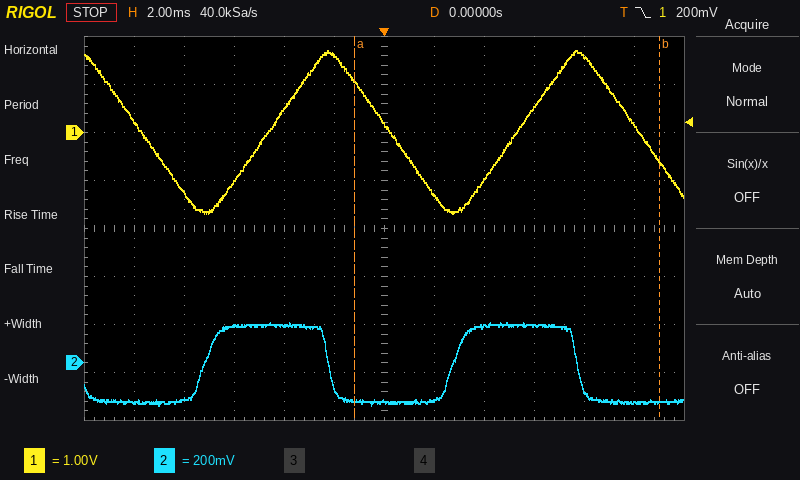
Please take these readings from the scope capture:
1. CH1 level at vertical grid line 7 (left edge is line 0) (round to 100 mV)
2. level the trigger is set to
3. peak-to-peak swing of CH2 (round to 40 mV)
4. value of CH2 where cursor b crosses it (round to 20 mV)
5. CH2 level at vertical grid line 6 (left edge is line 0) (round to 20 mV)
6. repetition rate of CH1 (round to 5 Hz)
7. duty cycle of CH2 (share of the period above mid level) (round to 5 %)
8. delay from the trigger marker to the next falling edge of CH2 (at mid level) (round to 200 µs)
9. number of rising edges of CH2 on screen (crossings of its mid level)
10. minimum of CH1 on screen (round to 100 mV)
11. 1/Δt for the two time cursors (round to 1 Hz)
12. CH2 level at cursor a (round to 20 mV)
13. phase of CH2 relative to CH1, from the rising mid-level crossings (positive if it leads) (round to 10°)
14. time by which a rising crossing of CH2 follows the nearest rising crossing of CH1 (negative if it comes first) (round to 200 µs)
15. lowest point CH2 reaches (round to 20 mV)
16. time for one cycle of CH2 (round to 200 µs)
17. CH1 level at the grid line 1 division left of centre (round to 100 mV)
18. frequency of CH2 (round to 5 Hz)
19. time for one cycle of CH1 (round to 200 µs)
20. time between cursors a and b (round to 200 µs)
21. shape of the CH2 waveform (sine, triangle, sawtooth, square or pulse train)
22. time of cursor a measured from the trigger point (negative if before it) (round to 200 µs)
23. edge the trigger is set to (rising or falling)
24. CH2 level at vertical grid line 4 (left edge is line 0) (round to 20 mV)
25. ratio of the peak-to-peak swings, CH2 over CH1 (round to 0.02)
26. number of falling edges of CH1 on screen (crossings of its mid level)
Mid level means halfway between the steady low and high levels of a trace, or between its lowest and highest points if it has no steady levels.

-1.3 V
200 mV
360 mV
-160 mV
-160 mV
100 Hz
50 %
7.8 ms
2
-1.7 V
82 Hz
-160 mV
+90°
-2.6 ms
-180 mV
10.0 ms
1.6 V
100 Hz
10.0 ms
12.2 ms
square
-1.2 ms
falling
160 mV
0.10
3
